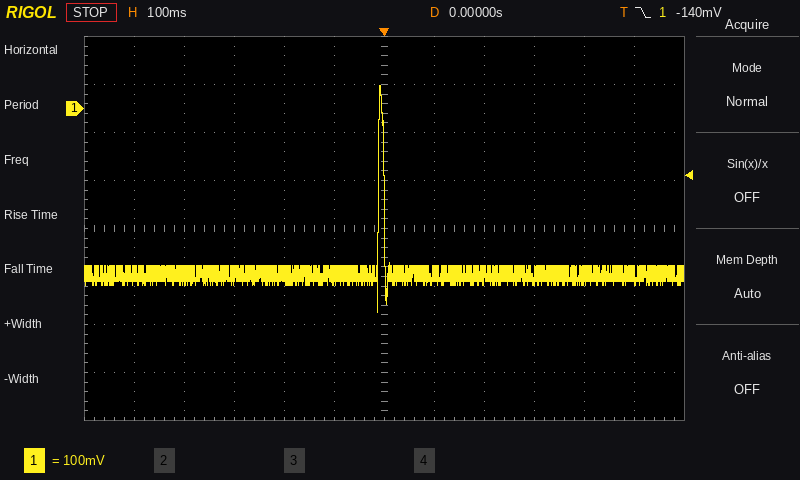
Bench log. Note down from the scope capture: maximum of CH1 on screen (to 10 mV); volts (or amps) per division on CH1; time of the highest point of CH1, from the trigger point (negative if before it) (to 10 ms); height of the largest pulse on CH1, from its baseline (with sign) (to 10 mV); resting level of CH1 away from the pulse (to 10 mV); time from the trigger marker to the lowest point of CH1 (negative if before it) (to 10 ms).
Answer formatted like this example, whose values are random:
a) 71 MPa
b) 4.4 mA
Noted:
a) 50 mV
b) 100 mV
c) -10 ms
d) +390 mV
e) -340 mV
f) -10 ms
